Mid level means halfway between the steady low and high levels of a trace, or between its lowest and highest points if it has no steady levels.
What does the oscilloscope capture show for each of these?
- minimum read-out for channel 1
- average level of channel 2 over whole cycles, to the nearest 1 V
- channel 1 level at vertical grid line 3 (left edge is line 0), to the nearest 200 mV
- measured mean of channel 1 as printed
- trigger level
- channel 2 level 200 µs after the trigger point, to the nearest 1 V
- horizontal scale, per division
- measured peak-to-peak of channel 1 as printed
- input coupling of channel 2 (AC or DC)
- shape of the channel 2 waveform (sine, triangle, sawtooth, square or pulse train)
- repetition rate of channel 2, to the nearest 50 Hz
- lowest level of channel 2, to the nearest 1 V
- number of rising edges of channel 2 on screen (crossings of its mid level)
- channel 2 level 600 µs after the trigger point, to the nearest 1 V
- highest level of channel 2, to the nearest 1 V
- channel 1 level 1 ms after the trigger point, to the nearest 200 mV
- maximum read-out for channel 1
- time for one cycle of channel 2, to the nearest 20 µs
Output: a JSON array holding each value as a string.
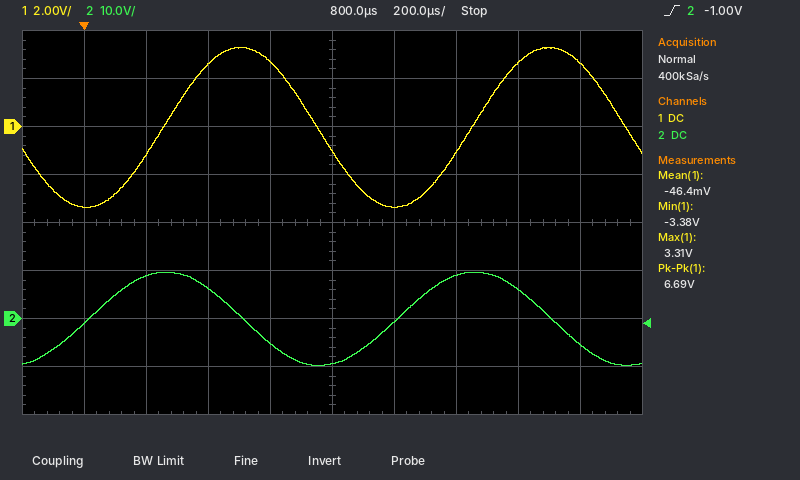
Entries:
["-3.38 V", "0 V", "2.6 V", "-46.4 mV", "-1.00 V", "9 V", "200 µs", "6.69 V", "DC", "sine", "1.00 kHz", "-10 V", "2", "-5 V", "10 V", "-3.4 V", "3.31 V", "1.00 ms"]
